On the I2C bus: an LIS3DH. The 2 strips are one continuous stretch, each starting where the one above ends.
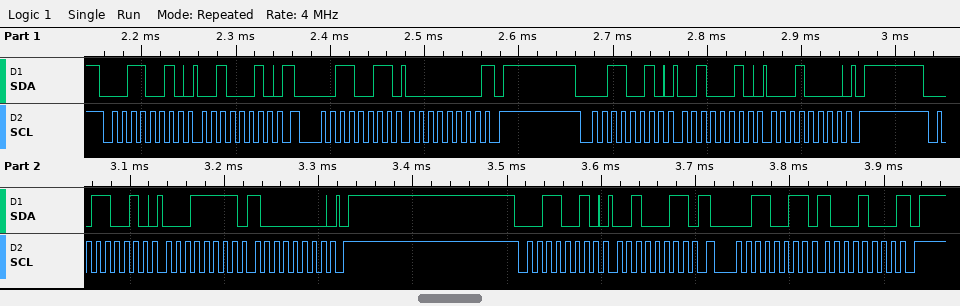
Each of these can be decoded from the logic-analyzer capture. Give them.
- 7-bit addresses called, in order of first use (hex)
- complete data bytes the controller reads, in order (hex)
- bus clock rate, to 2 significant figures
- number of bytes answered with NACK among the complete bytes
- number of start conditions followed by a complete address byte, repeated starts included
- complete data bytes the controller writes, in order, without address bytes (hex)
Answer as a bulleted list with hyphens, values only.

- 0x19
- 00 88
- 100 kHz
- 2
- 6
- 22 22 10 1F 80 23
